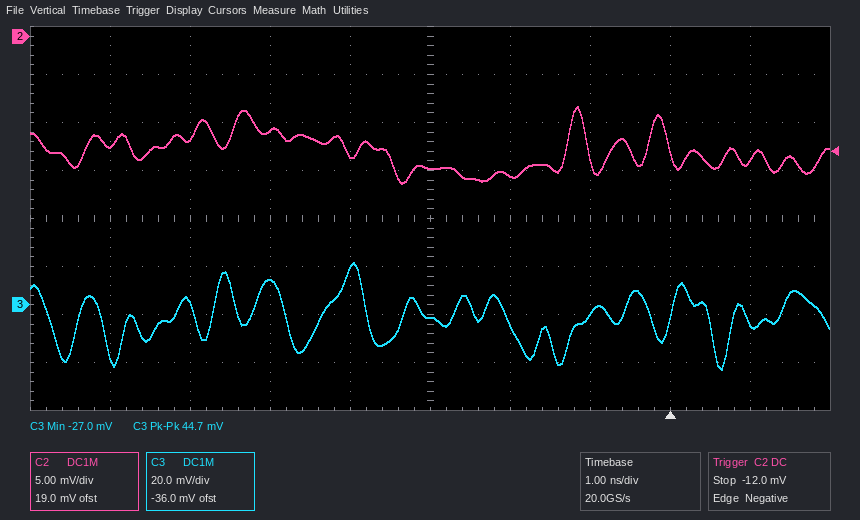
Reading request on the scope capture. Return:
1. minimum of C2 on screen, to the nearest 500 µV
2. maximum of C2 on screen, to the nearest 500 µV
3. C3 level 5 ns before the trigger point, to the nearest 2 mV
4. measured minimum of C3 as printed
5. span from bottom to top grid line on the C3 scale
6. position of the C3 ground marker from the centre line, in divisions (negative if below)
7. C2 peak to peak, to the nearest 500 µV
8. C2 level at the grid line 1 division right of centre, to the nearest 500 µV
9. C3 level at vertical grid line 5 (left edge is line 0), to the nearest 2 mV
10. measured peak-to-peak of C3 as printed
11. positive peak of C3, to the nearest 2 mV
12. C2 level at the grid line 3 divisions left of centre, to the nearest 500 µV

-15.5 mV
-7.5 mV
10 mV
-27.0 mV
160 mV
-1.8 div
8.0 mV
-14.5 mV
-6 mV
44.7 mV
18 mV
-10.5 mV
